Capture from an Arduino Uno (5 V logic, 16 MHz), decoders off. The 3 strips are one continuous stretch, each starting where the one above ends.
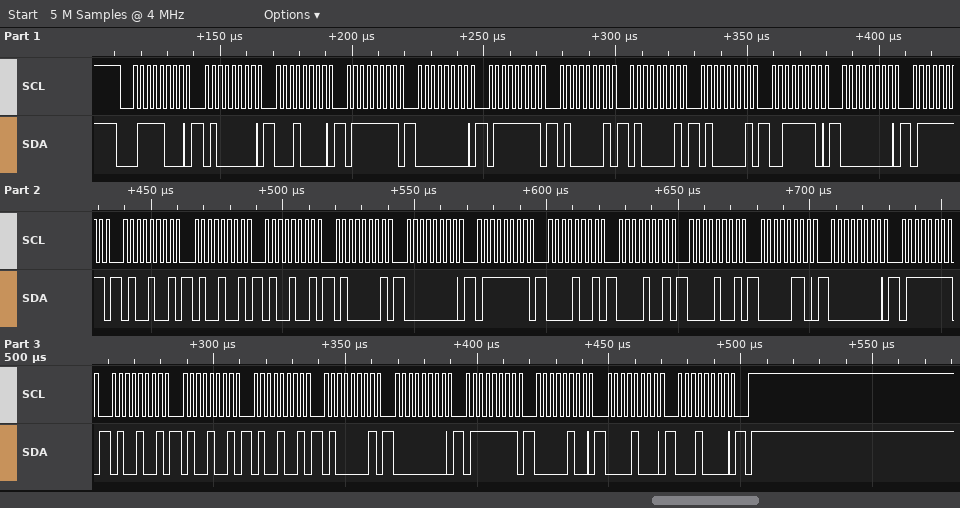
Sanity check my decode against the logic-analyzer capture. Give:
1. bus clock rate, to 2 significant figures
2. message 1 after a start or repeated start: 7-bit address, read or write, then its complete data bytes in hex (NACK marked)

400 kHz
0x3C write: 40 10 7F 00 7F 41 41 41 3E 00 7F 49 49 49 41 00 7F 09 09 09 06 00 7F 49 49 49 41 00 7F 04 08 10
